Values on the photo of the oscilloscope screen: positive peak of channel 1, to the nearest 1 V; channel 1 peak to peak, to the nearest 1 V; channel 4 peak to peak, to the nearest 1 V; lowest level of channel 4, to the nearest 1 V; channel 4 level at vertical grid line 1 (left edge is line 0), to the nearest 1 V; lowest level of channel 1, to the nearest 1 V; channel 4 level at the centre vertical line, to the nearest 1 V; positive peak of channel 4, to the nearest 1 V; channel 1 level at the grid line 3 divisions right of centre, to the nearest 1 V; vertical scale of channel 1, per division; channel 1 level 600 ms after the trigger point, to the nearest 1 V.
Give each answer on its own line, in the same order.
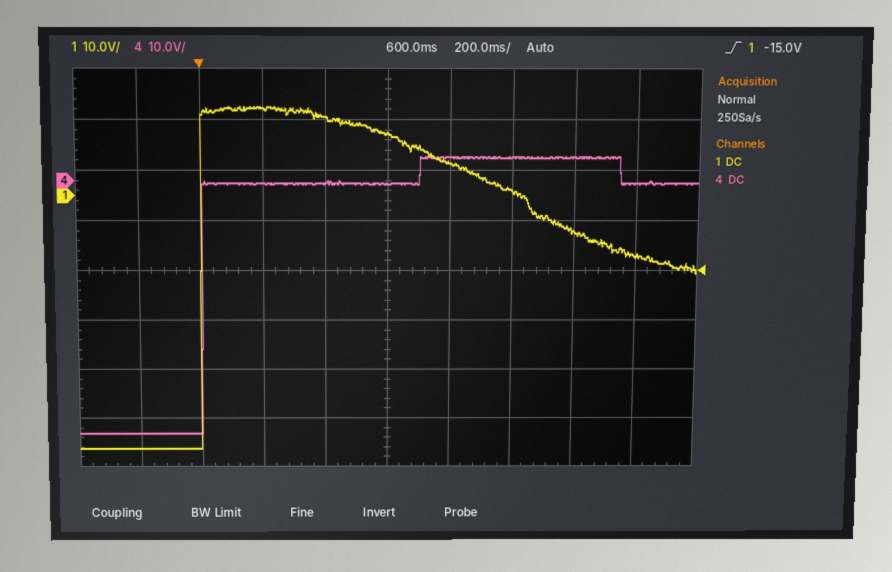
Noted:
18 V
69 V
56 V
-51 V
-51 V
-51 V
-1 V
5 V
-7 V
10 V
12 V
